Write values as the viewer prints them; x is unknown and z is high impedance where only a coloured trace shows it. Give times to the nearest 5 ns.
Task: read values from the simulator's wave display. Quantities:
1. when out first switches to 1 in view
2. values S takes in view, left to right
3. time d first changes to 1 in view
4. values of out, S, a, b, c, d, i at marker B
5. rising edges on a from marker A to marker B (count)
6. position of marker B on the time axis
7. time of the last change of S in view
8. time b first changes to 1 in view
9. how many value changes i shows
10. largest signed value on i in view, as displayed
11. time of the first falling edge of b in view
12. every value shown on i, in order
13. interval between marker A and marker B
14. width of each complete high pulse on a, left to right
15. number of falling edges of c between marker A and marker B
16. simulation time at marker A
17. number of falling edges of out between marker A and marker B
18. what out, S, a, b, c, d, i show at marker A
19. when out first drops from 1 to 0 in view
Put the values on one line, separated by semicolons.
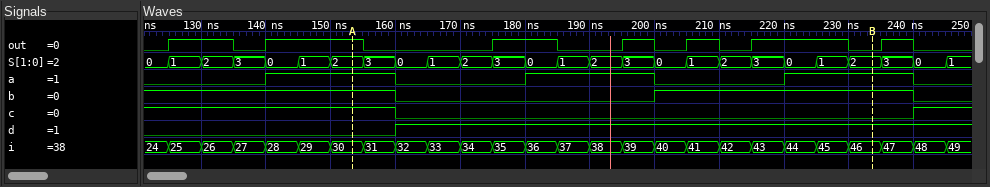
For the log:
125 ns; 0, 1, 2, 3, 0, 1, 2, 3, 0, 1, 2, 3, 0, 1, 2, 3, 0, 1, 2, 3, 0, 1, 2, 3, 0, 1; 160 ns; out=0, S=2, a=1, b=1, c=0, d=1, i=46; 2; 235 ns; 245 ns; 200 ns; 25; 49; 160 ns; 24, 25, 26, 27, 28, 29, 30, 31, 32, 33, 34, 35, 36, 37, 38, 39, 40, 41, 42, 43, 44, 45, 46, 47, 48, 49; 80 ns; 20 ns, 20 ns, 20 ns; 1; 155 ns; 5; out=1, S=2, a=1, b=1, c=1, d=0, i=30; 135 ns
